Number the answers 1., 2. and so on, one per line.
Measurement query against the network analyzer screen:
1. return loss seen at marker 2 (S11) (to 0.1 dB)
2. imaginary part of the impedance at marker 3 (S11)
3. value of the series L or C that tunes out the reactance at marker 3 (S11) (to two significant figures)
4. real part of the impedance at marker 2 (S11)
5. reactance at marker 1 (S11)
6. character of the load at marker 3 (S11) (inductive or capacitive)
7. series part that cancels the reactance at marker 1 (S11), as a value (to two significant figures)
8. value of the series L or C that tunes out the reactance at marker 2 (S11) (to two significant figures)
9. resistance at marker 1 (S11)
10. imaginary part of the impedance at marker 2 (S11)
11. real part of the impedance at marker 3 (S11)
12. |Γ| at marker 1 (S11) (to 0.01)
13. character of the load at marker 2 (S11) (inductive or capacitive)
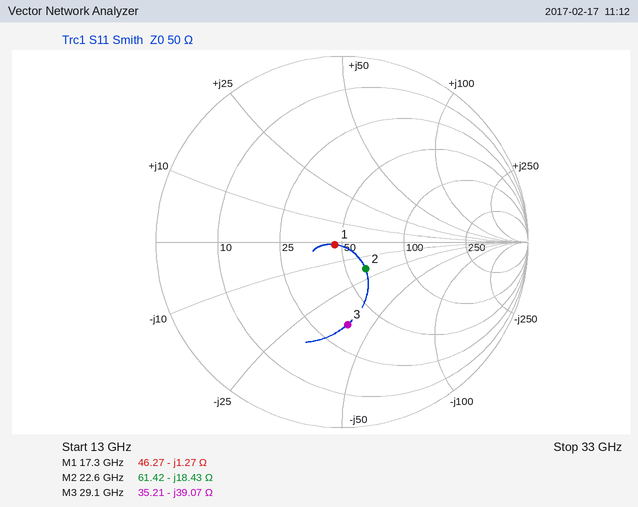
1. 14.3 dB
2. -39.07 Ω
3. 210 pH
4. 61.42 Ω
5. -1.27 Ω
6. capacitive
7. 12 pH
8. 130 pH
9. 46.27 Ω
10. -18.43 Ω
11. 35.21 Ω
12. 0.04
13. capacitive
